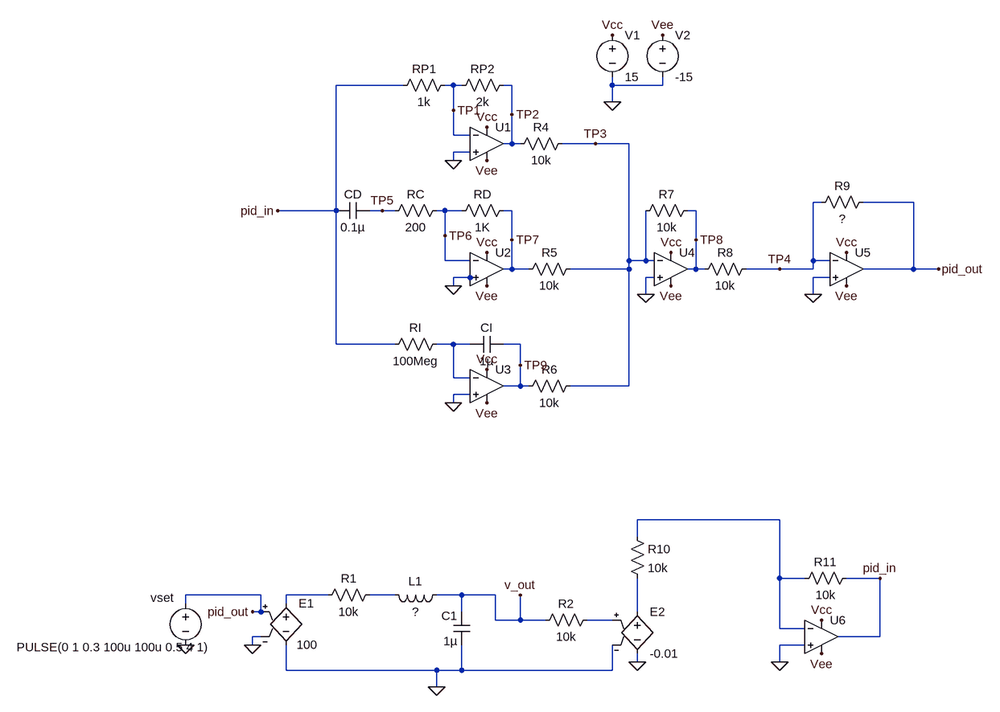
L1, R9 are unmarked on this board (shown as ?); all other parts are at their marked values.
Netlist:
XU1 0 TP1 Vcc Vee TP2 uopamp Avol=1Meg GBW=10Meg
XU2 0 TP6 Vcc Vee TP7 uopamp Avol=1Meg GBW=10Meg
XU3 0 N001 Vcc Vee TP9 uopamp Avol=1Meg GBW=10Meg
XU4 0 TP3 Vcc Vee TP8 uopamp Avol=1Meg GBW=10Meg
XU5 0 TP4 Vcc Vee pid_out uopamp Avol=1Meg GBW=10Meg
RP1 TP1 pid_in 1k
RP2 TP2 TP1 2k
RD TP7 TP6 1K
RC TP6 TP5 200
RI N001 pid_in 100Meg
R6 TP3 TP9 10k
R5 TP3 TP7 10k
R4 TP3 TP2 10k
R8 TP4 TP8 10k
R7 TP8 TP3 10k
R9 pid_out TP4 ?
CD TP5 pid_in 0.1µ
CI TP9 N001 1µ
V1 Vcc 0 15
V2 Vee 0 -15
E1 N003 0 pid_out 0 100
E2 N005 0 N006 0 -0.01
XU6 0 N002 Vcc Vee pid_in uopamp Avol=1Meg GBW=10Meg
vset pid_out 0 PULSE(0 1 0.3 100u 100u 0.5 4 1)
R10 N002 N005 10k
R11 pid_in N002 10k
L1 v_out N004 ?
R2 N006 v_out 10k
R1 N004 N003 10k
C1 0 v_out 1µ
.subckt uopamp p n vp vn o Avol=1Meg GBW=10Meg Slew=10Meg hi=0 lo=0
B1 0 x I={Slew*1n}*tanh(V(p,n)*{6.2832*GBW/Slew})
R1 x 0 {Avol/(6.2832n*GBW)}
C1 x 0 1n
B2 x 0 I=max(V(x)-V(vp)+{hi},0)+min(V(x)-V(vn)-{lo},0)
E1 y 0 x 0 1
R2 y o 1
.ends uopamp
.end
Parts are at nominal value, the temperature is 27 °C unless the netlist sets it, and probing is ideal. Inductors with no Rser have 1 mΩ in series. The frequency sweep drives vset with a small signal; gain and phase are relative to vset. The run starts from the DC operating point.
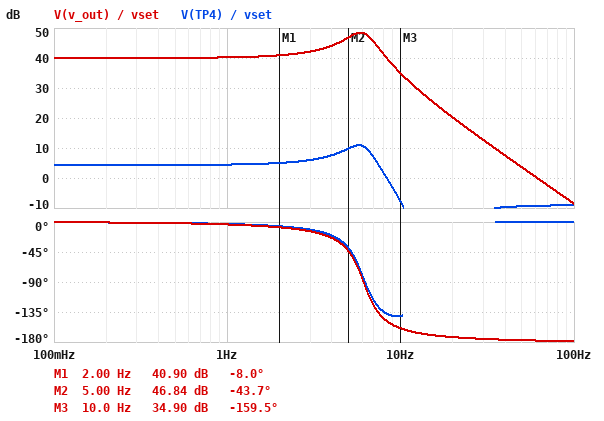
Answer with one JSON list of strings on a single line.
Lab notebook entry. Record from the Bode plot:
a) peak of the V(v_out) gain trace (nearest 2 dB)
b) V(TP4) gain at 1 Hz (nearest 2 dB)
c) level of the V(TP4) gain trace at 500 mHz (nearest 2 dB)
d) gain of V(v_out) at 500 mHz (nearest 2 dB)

["48 dB", "4 dB", "4 dB", "40 dB"]
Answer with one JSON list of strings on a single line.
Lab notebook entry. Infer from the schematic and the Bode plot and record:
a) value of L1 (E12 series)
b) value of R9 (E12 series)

["680 H", "18 kΩ"]
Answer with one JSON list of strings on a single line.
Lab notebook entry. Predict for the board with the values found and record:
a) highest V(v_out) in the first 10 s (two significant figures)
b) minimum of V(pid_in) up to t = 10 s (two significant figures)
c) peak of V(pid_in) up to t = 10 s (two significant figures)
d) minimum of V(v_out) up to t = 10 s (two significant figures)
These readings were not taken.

["150 V", "-530 mV", "1.5 V", "-53 V"]
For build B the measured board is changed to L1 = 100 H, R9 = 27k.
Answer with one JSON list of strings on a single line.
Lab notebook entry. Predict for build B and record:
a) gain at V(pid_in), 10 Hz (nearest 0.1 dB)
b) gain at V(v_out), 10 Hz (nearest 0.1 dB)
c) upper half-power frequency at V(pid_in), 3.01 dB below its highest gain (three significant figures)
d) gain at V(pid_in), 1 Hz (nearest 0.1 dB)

["1.2 dB", "41.2 dB", "18.6 Hz", "0 dB"]
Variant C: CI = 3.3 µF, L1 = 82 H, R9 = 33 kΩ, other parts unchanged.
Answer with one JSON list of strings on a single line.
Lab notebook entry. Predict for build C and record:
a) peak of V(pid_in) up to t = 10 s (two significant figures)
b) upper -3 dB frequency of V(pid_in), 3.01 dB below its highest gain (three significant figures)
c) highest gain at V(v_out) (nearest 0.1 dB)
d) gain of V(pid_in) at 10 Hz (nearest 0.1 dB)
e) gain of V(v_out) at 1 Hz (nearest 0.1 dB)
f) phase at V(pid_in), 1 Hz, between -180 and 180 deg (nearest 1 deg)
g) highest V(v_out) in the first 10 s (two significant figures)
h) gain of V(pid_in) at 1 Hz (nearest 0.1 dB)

["1.1 V", "20.1 Hz", "40.7 dB", "0.7 dB", "40.0 dB", "-4 deg", "110 V", "0 dB"]
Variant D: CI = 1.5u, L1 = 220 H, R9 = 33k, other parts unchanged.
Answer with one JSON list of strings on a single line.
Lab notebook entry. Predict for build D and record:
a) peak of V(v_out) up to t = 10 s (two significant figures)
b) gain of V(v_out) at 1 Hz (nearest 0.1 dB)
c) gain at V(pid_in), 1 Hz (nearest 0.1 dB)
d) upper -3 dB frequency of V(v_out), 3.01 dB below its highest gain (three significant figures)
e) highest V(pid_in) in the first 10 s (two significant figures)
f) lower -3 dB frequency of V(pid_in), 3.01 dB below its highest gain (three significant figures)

["130 V", "40.1 dB", "0.1 dB", "12.7 Hz", "1.3 V", "3.99 Hz"]
